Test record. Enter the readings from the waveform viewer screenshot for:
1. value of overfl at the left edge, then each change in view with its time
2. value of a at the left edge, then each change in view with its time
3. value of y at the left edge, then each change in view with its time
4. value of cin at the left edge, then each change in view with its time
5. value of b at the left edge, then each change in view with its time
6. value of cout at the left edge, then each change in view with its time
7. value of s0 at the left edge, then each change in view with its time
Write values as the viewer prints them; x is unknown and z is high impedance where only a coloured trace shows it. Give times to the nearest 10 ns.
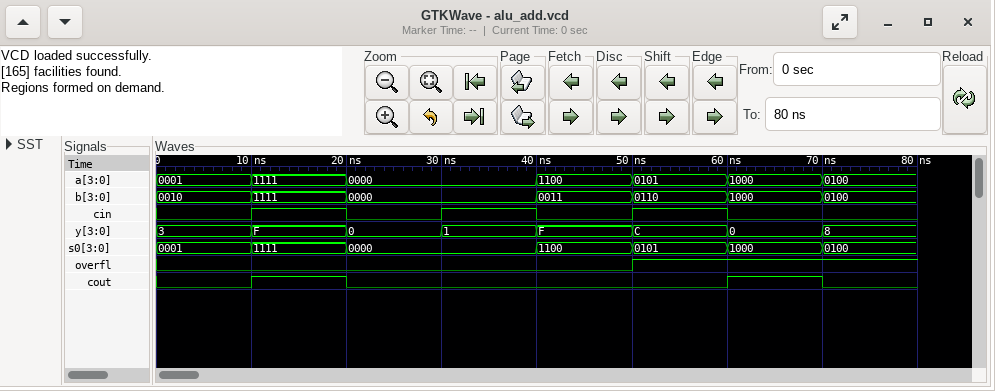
0, 1 at 50 ns
0001, 1111 at 10 ns, 0000 at 20 ns, 1100 at 40 ns, 0101 at 50 ns, 1000 at 60 ns, 0100 at 70 ns
3, F at 10 ns, 0 at 20 ns, 1 at 30 ns, F at 40 ns, C at 50 ns, 0 at 60 ns, 8 at 70 ns
0, 1 at 10 ns, 0 at 20 ns, 1 at 30 ns, 0 at 40 ns, 1 at 50 ns, 0 at 60 ns
0010, 1111 at 10 ns, 0000 at 20 ns, 0011 at 40 ns, 0110 at 50 ns, 1000 at 60 ns, 0100 at 70 ns
0, 1 at 10 ns, 0 at 20 ns, 1 at 60 ns, 0 at 70 ns
0001, 1111 at 10 ns, 0000 at 20 ns, 1100 at 40 ns, 0101 at 50 ns, 1000 at 60 ns, 0100 at 70 ns
